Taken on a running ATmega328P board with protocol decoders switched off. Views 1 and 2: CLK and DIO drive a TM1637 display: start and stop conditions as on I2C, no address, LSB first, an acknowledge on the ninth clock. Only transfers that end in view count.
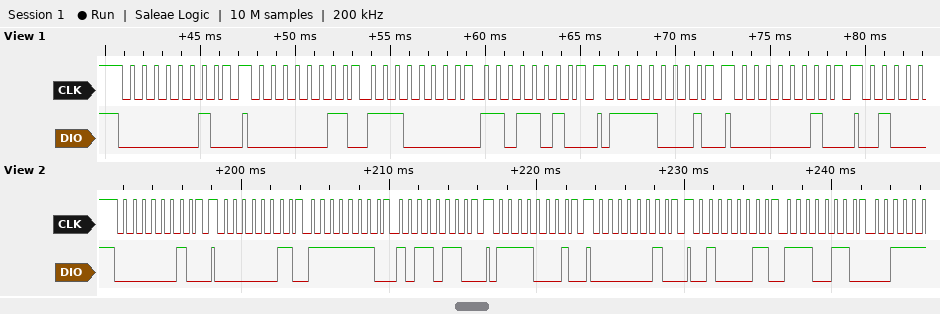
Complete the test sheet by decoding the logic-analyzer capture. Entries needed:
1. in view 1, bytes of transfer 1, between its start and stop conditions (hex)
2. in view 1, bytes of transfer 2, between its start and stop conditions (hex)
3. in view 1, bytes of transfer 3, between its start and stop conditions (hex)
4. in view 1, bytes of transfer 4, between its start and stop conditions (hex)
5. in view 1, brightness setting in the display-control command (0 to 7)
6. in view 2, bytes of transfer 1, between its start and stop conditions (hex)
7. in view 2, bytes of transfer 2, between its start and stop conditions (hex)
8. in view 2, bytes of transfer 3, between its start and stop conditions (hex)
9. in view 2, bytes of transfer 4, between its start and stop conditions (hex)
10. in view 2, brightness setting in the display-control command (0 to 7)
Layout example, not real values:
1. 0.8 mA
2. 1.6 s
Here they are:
1. 40
2. C0 07 5B
3. 8F
4. 40
5. 7
6. 40
7. C0 7F 6D
8. 8F
9. 40
10. 7
